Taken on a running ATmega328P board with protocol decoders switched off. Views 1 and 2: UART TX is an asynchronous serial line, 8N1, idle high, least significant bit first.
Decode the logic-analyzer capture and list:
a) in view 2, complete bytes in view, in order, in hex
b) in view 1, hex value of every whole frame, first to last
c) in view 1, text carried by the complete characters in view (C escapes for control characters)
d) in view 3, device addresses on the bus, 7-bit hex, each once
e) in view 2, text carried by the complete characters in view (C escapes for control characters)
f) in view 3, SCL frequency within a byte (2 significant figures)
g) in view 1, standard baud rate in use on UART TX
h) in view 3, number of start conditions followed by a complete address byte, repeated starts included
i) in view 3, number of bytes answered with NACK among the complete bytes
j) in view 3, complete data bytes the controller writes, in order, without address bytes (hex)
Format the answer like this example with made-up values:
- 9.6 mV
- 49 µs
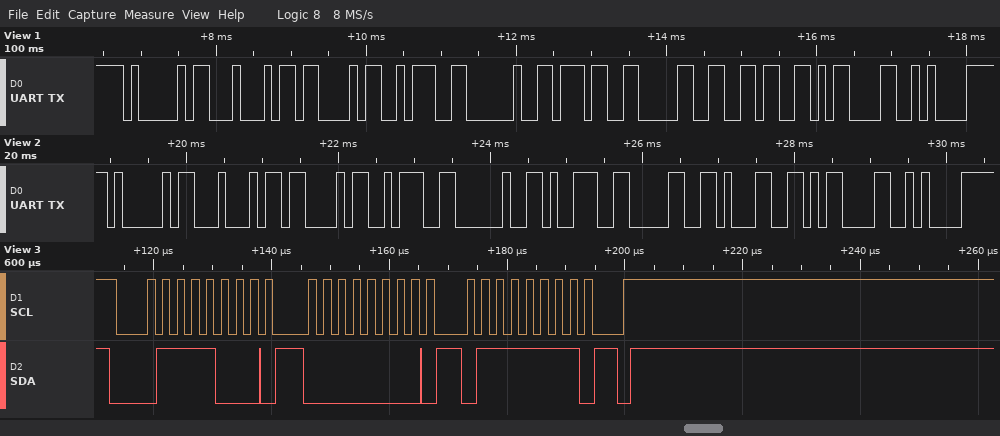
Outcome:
- 0x41 0x44 0x43 0x3A 0x20 0x39 0x30 0x31 0x0D 0x0A
- 0x41 0x44 0x43 0x3A 0x20 0x37 0x30 0x36 0x0D 0x0A
- "ADC: 706\r\n"
- 0x3C
- "ADC: 901\r\n"
- 400 kHz
- 9600 baud
- 1
- 0
- 00 7F
